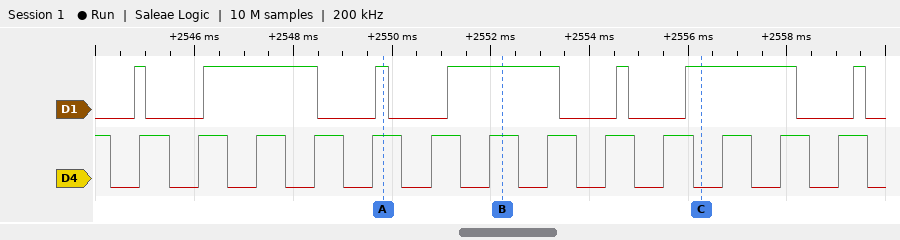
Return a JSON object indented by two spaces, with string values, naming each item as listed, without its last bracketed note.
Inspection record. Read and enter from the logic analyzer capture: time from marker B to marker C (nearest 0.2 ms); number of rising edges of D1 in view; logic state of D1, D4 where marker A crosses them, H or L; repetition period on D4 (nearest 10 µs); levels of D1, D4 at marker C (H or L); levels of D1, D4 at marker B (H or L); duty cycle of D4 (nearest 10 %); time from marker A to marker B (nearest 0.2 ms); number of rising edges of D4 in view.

{
  "time from marker B to marker C": "4 ms",
  "number of rising edges of D1 in view": "7",
  "logic state of D1, D4 where marker A crosses them, H or L": "D1=H, D4=H",
  "repetition period on D4": "1180 µs",
  "levels of D1, D4 at marker C": "D1=H, D4=L",
  "levels of D1, D4 at marker B": "D1=H, D4=H",
  "duty cycle of D4": "50 %",
  "time from marker A to marker B": "2.4 ms",
  "number of rising edges of D4 in view": "13"
}
